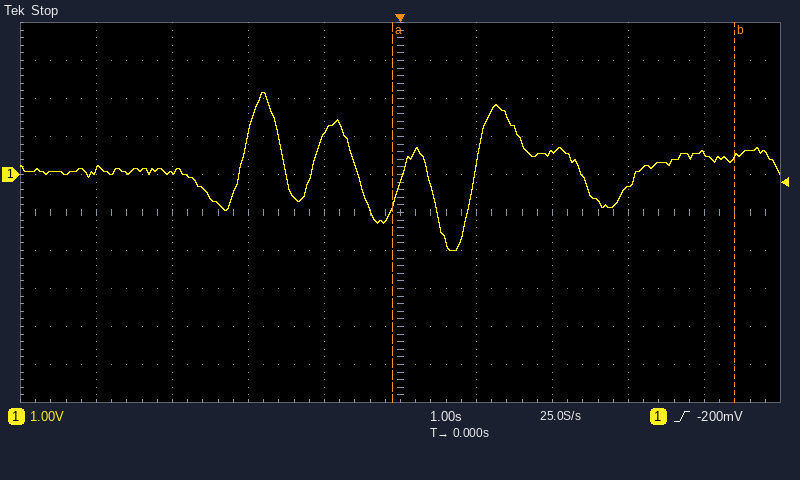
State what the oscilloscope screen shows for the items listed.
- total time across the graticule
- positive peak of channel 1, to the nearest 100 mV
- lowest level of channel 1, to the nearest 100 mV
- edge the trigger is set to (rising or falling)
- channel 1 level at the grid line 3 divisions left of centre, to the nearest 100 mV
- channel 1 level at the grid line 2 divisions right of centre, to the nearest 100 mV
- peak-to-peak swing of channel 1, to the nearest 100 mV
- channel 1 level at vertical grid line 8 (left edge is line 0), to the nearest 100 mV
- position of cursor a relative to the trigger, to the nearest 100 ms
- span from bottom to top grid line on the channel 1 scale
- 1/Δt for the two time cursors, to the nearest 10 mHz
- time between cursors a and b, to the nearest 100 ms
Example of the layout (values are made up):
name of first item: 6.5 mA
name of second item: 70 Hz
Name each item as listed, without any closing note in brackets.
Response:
total time across the graticule: 10 s
positive peak of channel 1, to the nearest 100 mV: 2.2 V
lowest level of channel 1, to the nearest 100 mV: -2.0 V
edge the trigger is set to: rising
channel 1 level at the grid line 3 divisions left of centre, to the nearest 100 mV: 100 mV
channel 1 level at the grid line 2 divisions right of centre, to the nearest 100 mV: 600 mV
peak-to-peak swing of channel 1, to the nearest 100 mV: 4.2 V
channel 1 level at vertical grid line 8 (left edge is line 0), to the nearest 100 mV: -300 mV
position of cursor a relative to the trigger, to the nearest 100 ms: -100 ms
span from bottom to top grid line on the channel 1 scale: 10 V
1/Δt for the two time cursors, to the nearest 10 mHz: 220 mHz
time between cursors a and b, to the nearest 100 ms: 4.5 s
